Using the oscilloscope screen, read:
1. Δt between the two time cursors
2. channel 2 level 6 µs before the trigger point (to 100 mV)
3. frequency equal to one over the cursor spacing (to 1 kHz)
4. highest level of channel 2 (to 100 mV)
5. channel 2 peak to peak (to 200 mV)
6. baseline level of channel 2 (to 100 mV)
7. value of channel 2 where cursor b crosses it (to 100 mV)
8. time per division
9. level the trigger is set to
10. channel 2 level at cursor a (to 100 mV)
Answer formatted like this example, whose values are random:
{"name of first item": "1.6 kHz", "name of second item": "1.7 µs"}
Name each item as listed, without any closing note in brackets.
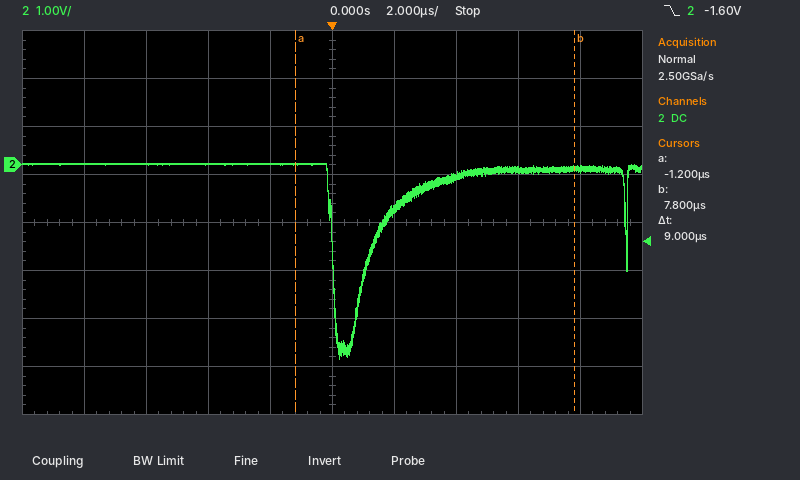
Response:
{"Δt between the two time cursors": "9 µs", "channel 2 level 6 µs before the trigger point": "0.0 V", "frequency equal to one over the cursor spacing": "111 kHz", "highest level of channel 2": "0.0 V", "channel 2 peak to peak": "4.0 V", "baseline level of channel 2": "0.0 V", "value of channel 2 where cursor b crosses it": "-100 mV", "time per division": "2 µs", "level the trigger is set to": "-1.60 V", "channel 2 level at cursor a": "0.0 V"}
